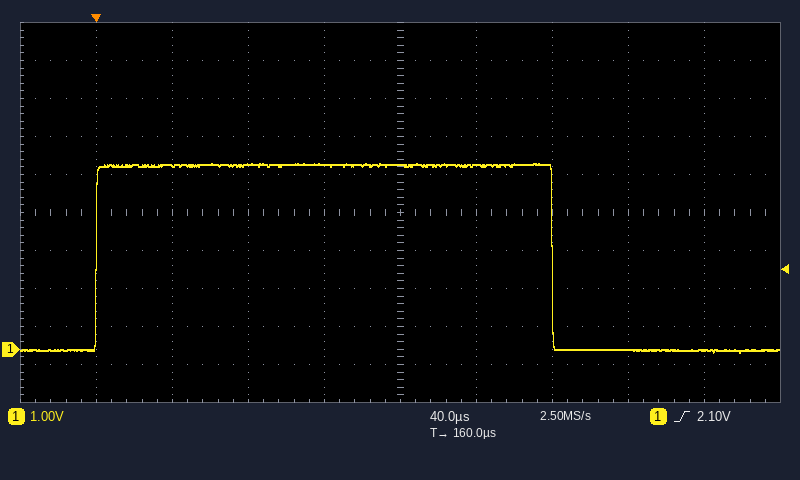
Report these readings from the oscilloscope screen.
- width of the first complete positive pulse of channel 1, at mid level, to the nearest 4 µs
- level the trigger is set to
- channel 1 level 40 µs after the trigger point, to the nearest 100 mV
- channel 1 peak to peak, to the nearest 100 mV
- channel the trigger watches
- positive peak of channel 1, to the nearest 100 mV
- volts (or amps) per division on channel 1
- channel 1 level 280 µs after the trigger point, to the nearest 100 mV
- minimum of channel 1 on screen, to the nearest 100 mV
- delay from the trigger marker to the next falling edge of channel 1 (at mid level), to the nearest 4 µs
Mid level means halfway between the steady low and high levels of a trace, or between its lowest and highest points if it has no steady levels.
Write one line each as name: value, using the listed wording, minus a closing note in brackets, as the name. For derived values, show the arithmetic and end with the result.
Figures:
width of the first complete positive pulse of channel 1, at mid level, to the nearest 4 µs: 240 µs
level the trigger is set to: 2.10 V
channel 1 level 40 µs after the trigger point, to the nearest 100 mV: 4.8 V
channel 1 peak to peak, to the nearest 100 mV: 4.9 V − (-100 mV) = 5.0 V
channel the trigger watches: channel 1
positive peak of channel 1, to the nearest 100 mV: 4.9 V
volts (or amps) per division on channel 1: 1 V
channel 1 level 280 µs after the trigger point, to the nearest 100 mV: 0.0 V
minimum of channel 1 on screen, to the nearest 100 mV: -100 mV
delay from the trigger marker to the next falling edge of channel 1 (at mid level), to the nearest 4 µs: 240 µs
